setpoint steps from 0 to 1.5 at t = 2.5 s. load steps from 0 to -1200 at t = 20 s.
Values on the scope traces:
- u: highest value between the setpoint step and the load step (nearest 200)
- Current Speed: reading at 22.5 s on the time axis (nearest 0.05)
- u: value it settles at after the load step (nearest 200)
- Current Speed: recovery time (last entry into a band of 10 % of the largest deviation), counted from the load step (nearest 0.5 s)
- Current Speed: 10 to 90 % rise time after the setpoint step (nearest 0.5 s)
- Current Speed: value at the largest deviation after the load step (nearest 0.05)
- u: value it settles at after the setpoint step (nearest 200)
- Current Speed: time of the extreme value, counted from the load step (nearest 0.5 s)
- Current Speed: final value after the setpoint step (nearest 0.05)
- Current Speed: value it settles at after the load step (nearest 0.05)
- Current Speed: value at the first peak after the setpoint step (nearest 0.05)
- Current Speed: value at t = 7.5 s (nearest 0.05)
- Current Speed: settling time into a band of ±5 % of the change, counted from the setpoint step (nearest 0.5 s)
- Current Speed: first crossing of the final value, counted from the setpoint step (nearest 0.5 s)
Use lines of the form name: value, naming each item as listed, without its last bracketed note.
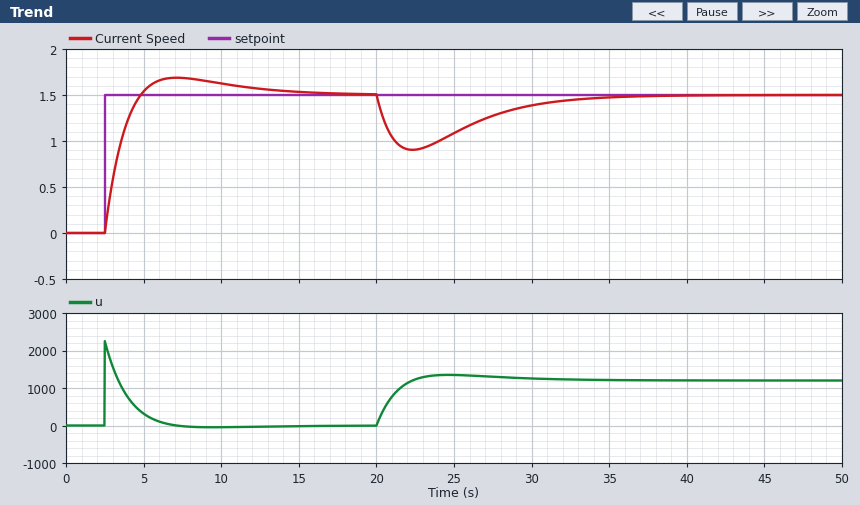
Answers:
u: highest value between the setpoint step and the load step: 2200
Current Speed: reading at 22.5 s on the time axis: 0.90
u: value it settles at after the load step: 1200
Current Speed: recovery time (last entry into a band of 10 % of the largest deviation), counted from the load step: 12.0 s
Current Speed: 10 to 90 % rise time after the setpoint step: 1.5 s
Current Speed: value at the largest deviation after the load step: 0.90
u: value it settles at after the setpoint step: 0
Current Speed: time of the extreme value, counted from the load step: 2.5 s
Current Speed: final value after the setpoint step: 1.50
Current Speed: value it settles at after the load step: 1.50
Current Speed: value at the first peak after the setpoint step: 1.70
Current Speed: value at t = 7.5 s: 1.70
Current Speed: settling time into a band of ±5 % of the change, counted from the setpoint step: 9.5 s
Current Speed: first crossing of the final value, counted from the setpoint step: 2.5 s
